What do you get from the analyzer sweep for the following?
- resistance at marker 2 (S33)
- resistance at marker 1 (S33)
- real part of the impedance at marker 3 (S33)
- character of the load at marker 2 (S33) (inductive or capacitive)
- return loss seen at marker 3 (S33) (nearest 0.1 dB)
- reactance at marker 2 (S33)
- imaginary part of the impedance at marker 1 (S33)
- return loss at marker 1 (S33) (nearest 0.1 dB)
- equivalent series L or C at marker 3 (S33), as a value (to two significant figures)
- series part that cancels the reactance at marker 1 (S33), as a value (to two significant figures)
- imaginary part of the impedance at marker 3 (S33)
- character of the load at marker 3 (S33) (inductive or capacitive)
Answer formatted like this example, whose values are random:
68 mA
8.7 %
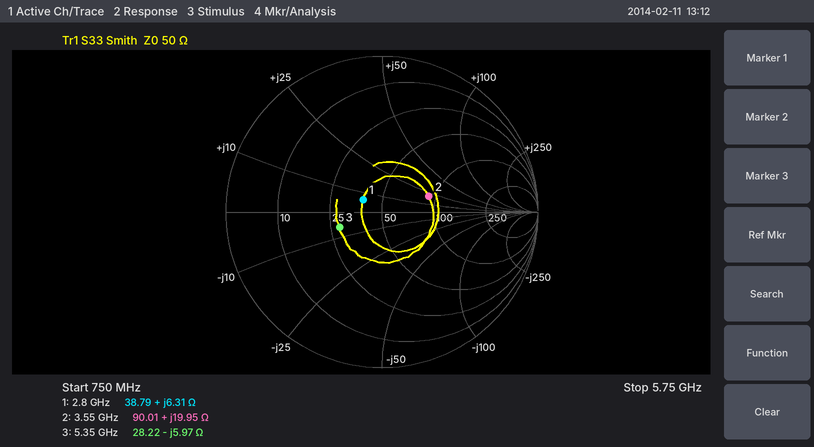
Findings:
90.01 Ω
38.79 Ω
28.22 Ω
inductive
10.8 dB
+19.95 Ω
+6.31 Ω
16.8 dB
5.0 pF
9.0 pF
-5.97 Ω
capacitive
